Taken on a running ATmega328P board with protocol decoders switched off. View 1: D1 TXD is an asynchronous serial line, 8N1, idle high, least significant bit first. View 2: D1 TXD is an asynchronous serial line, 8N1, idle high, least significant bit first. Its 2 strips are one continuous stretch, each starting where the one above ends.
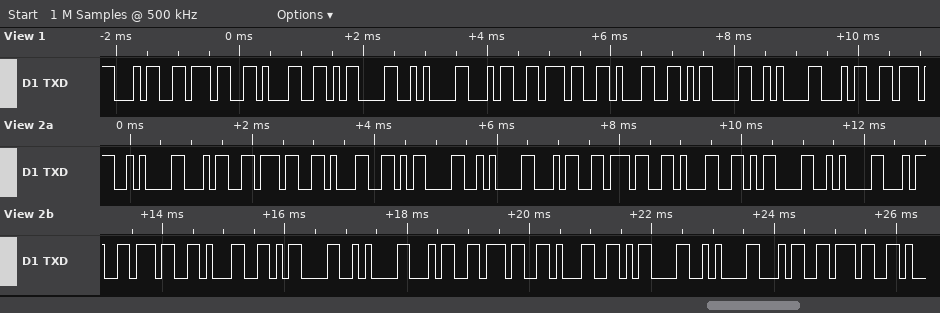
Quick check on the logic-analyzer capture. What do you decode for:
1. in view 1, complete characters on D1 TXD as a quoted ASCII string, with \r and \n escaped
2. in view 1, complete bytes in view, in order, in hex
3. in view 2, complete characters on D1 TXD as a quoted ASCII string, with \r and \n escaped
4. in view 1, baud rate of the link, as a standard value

"471\r\n471\r\n4"
34 37 31 0D 0A 34 37 31 0D 0A 34
"\n471\r\n471\r\n471\r\n471\r\n47"
9600 baud
